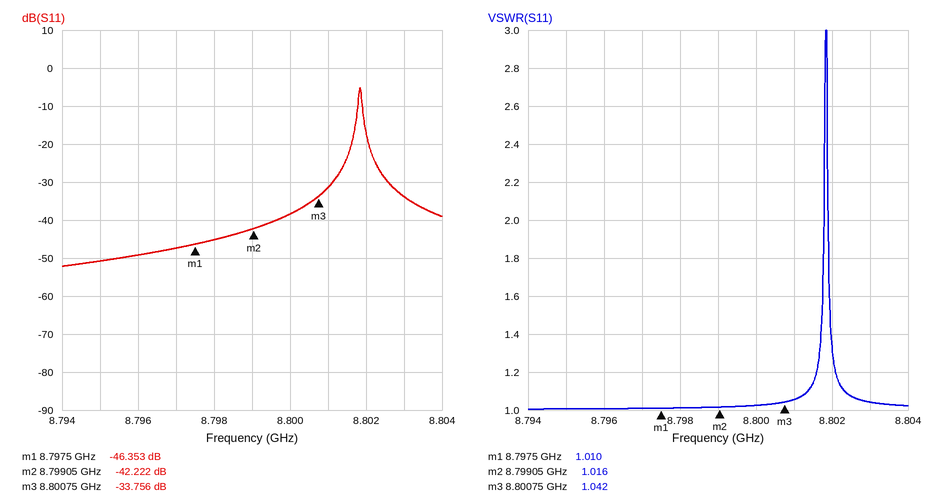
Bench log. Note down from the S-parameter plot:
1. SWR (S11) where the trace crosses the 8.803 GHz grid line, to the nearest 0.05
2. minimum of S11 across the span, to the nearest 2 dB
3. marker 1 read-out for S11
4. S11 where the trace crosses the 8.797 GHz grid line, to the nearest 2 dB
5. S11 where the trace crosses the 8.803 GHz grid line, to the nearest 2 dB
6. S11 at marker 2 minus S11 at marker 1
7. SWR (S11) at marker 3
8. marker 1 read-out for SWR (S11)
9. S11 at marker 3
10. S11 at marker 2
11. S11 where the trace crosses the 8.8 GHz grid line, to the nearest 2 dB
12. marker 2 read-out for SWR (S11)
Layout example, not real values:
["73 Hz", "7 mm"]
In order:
["1.05", "-52 dB", "-46.353 dB", "-48 dB", "-34 dB", "4.131 dB", "1.042", "1.010", "-33.756 dB", "-42.222 dB", "-38 dB", "1.016"]
